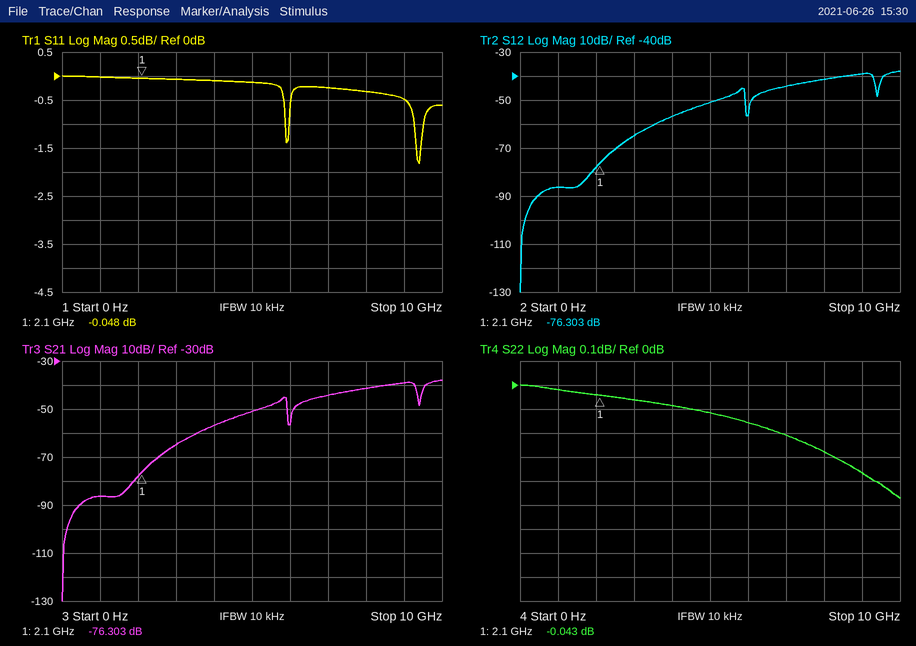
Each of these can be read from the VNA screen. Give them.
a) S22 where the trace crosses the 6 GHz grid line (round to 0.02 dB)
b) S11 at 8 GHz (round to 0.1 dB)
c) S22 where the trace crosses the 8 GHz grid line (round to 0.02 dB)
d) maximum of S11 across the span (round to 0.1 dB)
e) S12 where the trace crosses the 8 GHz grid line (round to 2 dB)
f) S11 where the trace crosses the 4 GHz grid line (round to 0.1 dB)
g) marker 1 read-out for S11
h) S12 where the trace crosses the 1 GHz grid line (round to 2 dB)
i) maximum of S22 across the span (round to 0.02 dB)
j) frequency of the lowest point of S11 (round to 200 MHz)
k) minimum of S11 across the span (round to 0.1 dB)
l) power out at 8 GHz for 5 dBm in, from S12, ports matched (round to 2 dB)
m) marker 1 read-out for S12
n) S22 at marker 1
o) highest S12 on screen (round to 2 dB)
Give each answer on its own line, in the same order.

-0.16 dB
-0.3 dB
-0.28 dB
0.0 dB
-42 dB
-0.1 dB
-0.048 dB
-86 dB
0.00 dB
9.4 GHz
-1.8 dB
-36 dBm
-76.303 dB
-0.043 dB
-38 dB
